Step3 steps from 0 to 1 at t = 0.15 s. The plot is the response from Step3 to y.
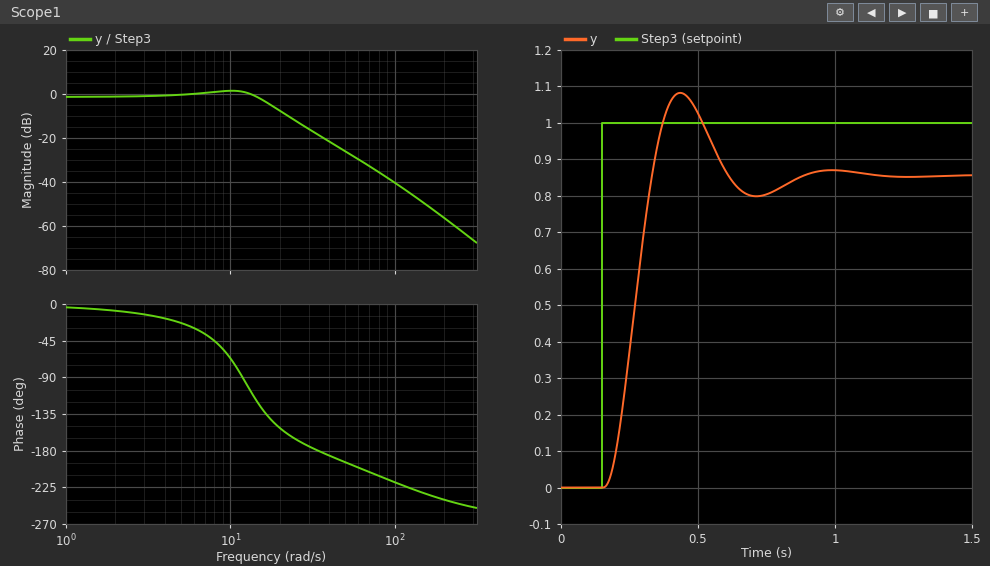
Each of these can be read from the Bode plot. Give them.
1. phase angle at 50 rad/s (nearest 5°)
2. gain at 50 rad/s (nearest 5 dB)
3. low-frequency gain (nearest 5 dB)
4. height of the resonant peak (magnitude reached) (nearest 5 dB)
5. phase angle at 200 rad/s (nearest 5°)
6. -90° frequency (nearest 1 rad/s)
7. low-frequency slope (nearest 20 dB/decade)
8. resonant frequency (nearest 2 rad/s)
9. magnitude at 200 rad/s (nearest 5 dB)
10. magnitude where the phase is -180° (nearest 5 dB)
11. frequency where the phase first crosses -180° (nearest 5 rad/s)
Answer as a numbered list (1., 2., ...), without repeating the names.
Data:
1. -195°
2. -25 dB
3. 0 dB
4. 0 dB
5. -240°
6. 12 rad/s
7. 0 dB/decade
8. 10 rad/s
9. -55 dB
10. -20 dB
11. 35 rad/s
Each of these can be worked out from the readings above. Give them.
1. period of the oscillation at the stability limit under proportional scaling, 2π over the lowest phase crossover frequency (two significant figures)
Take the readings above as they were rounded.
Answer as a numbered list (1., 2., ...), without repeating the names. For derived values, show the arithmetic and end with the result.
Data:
1. 2π / 35 = 0.18 s
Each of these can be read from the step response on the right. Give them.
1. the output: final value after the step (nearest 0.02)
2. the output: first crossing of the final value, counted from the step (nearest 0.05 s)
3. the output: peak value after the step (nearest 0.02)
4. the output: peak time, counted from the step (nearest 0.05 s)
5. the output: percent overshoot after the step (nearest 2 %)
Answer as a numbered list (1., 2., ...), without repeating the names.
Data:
1. 0.86
2. 0.20 s
3. 1.08
4. 0.30 s
5. 26 %
